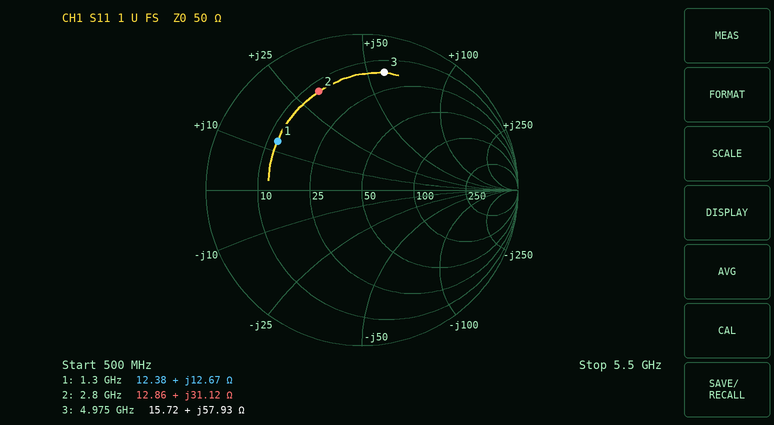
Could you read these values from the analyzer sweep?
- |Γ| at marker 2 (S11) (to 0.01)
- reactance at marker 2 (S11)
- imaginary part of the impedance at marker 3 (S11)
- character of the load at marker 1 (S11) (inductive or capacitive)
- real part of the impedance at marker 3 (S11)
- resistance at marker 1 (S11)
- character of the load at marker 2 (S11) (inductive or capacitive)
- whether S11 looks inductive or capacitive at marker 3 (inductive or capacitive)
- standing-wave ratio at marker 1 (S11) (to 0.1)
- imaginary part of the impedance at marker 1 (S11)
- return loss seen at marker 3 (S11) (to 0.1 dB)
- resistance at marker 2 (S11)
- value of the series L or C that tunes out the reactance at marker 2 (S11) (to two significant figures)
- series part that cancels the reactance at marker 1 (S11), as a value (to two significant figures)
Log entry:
0.69
+31.12 Ω
+57.93 Ω
inductive
15.72 Ω
12.38 Ω
inductive
inductive
4.3
+12.67 Ω
2.3 dB
12.86 Ω
1.8 pF
9.7 pF
